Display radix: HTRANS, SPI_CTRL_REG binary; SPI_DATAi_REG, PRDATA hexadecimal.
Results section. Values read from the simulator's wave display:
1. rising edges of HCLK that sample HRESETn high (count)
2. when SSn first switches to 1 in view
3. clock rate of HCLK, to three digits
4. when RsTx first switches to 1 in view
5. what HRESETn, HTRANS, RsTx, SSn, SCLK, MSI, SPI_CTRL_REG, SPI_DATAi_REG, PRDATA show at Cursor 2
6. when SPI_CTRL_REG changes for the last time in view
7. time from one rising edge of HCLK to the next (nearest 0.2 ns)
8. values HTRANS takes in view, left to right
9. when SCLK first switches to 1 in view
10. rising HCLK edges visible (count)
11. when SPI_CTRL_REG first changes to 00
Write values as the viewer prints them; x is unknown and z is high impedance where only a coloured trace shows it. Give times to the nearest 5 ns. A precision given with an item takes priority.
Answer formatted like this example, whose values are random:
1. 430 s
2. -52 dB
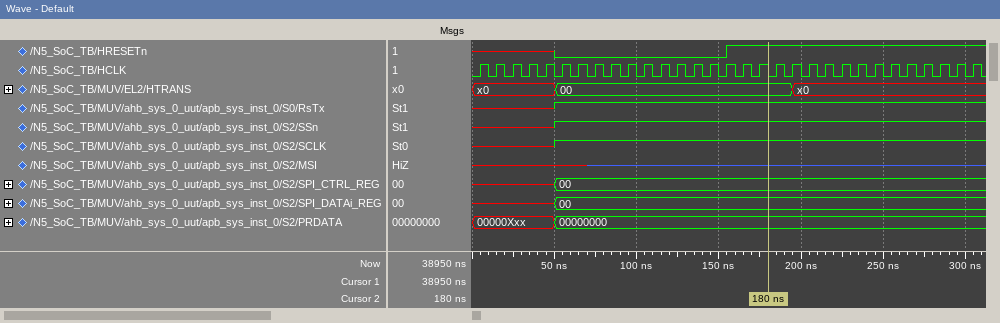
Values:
1. 15
2. 50 ns
3. 100 MHz
4. 50 ns
5. HRESETn=1, HTRANS=00, RsTx=1, SSn=1, SCLK=1, MSI=z, SPI_CTRL_REG=00, SPI_DATAi_REG=00, PRDATA=00000000
6. 50 ns
7. 10 ns
8. x0, 00, x0
9. 50 ns
10. 31
11. 50 ns
